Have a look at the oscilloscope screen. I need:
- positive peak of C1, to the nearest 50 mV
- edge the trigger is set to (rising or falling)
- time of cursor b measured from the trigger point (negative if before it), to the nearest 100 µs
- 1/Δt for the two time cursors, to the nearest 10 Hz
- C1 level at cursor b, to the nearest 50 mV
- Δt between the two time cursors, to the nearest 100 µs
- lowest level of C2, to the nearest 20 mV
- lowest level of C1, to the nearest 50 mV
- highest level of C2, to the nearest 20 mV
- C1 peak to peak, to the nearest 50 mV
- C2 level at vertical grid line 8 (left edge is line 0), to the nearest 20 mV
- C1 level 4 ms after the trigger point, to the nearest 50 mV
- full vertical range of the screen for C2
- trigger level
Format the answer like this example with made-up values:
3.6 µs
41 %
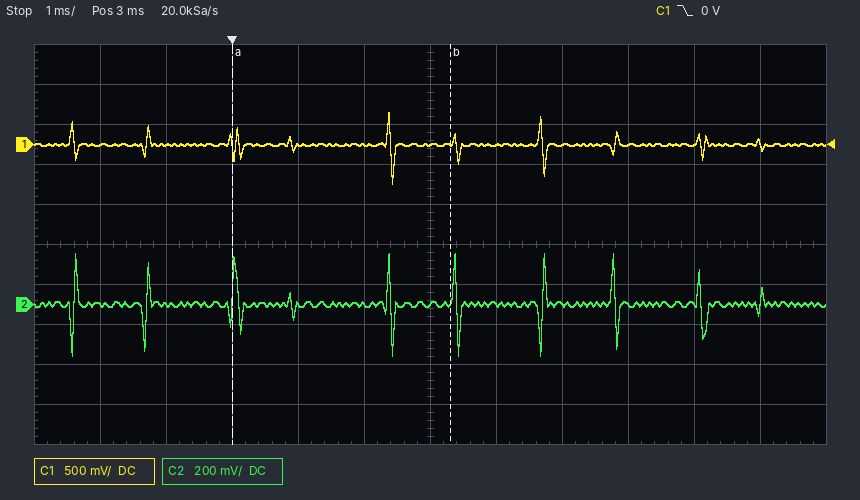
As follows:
400 mV
falling
+3.3 ms
300 Hz
50 mV
3.3 ms
-260 mV
-500 mV
260 mV
900 mV
0 mV
0 mV
2 V
0 V
